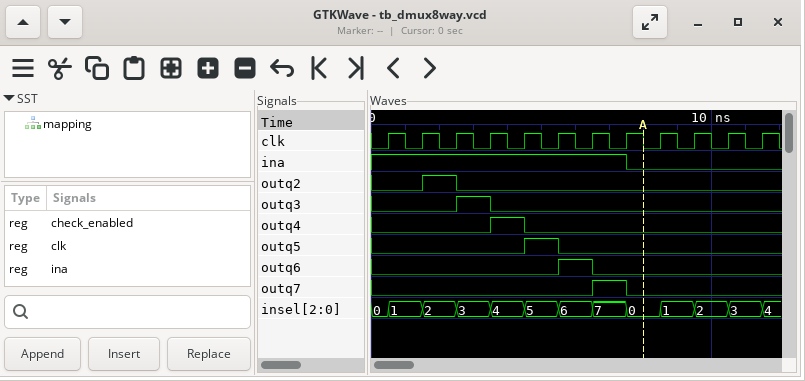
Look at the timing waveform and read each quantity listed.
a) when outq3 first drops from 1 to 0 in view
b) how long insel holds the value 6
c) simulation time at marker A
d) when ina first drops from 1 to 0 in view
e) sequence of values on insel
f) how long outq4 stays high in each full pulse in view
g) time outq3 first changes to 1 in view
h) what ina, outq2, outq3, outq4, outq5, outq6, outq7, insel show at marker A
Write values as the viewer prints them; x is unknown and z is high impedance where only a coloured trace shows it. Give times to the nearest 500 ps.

3500 ps
1000 ps
8000 ps
7500 ps
0, 1, 2, 3, 4, 5, 6, 7, 0, 1, 2, 3, 4
1000 ps
2500 ps
ina=0, outq2=0, outq3=0, outq4=0, outq5=0, outq6=0, outq7=0, insel=0
